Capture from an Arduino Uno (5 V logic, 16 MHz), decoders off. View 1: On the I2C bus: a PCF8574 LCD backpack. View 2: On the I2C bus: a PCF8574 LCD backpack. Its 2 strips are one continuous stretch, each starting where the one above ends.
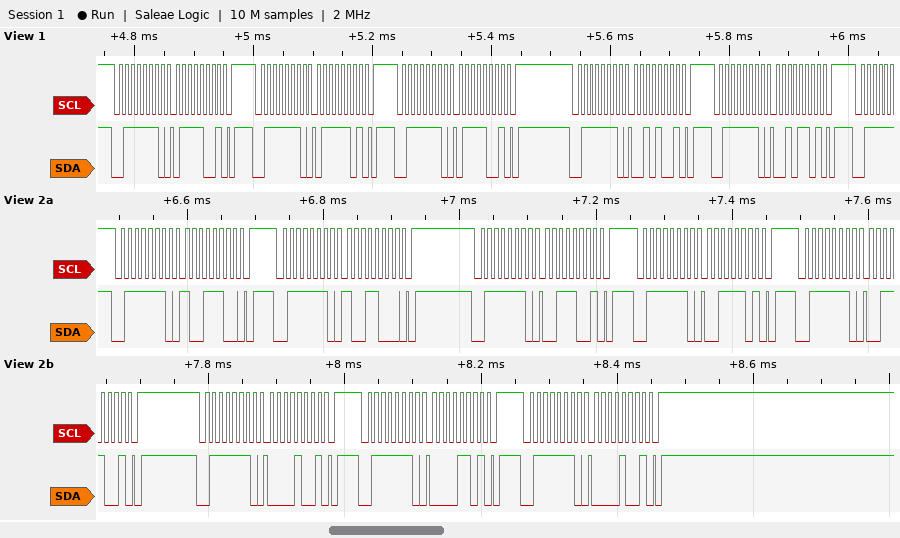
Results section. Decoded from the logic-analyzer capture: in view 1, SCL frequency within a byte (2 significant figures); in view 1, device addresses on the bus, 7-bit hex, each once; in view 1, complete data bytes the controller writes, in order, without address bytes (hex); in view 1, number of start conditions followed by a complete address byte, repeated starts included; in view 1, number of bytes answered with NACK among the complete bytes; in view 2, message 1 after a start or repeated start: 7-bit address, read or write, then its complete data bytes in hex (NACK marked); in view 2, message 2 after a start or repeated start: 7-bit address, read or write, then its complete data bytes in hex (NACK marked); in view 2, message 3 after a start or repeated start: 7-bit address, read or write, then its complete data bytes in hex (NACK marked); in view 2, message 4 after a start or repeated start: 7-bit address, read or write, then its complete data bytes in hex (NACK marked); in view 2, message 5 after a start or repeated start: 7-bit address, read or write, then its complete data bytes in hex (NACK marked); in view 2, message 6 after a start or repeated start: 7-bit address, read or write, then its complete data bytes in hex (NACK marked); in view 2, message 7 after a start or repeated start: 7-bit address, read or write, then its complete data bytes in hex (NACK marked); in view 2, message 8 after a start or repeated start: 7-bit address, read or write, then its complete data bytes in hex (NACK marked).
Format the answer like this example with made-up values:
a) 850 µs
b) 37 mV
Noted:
a) 100 kHz
b) 0x3F
c) 79 7D 79 29 2D
d) 5
e) 0
f) 0x3F write: 9C
g) 0x3F write: 98
h) 0x3F write: 39
i) 0x3F write: 3D
j) 0x3F write: 39
k) 0x3F write: 09
l) 0x3F write: 0D
m) 0x3F write: 09
